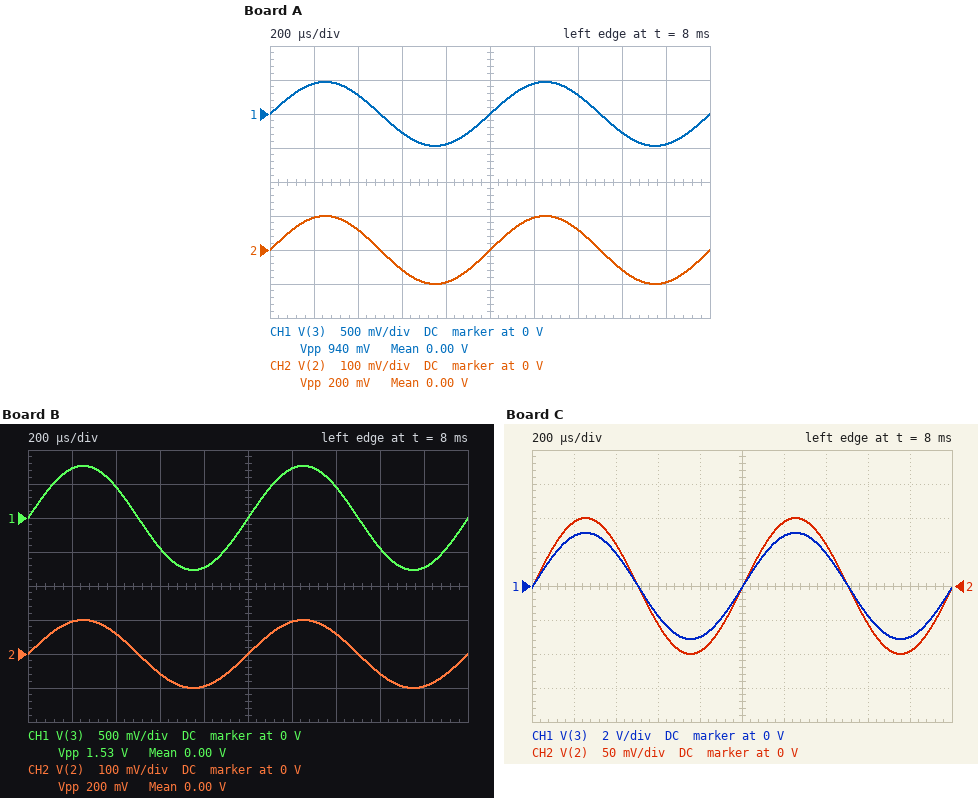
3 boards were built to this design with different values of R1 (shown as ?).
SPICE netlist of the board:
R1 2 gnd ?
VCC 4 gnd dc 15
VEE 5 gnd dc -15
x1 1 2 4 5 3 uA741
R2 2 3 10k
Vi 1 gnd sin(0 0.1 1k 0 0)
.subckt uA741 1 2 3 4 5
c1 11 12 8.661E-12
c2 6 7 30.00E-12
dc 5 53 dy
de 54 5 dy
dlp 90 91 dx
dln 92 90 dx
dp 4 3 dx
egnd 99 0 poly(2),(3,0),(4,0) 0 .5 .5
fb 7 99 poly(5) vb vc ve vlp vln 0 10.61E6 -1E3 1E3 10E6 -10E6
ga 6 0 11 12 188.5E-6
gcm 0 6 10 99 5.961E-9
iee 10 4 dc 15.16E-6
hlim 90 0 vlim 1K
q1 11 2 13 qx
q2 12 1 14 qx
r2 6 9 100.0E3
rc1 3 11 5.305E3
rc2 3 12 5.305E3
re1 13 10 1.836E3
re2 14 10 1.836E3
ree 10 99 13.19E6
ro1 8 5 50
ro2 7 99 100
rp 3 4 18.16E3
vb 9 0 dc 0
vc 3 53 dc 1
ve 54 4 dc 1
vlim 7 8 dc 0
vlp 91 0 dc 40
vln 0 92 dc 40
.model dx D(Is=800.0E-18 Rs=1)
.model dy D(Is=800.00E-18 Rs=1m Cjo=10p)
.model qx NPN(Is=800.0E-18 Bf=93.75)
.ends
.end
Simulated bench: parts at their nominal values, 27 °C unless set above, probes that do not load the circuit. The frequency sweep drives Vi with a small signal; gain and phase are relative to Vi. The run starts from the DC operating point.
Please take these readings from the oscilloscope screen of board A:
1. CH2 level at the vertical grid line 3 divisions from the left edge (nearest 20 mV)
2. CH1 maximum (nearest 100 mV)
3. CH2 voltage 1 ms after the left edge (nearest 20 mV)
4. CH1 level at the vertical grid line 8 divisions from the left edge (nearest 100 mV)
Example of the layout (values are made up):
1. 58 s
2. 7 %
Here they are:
1. -60 mV
2. 500 mV
3. 0 V
4. -300 mV
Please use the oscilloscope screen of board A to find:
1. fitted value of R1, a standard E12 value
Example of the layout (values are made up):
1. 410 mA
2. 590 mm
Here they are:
1. 2.7 kΩ
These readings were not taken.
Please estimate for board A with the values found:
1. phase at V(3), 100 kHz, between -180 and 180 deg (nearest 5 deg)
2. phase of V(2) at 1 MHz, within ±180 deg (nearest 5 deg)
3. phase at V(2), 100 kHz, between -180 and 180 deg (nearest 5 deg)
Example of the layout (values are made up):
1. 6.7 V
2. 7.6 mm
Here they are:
1. -25 deg
2. -110 deg
3. -25 deg
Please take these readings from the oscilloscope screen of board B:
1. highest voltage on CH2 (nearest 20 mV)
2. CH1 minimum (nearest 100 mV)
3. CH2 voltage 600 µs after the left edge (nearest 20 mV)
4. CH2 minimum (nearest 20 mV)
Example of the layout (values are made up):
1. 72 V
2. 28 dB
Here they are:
1. 100 mV
2. -800 mV
3. -60 mV
4. -100 mV
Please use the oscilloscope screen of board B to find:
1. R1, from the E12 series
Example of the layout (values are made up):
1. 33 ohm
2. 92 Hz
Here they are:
1. 1.5 kΩ
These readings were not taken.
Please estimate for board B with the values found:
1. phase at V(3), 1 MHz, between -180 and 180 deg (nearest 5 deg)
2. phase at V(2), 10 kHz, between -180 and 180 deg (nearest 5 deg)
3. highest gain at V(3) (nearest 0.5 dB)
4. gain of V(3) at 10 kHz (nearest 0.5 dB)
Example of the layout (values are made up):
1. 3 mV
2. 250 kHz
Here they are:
1. -115 deg
2. -5 deg
3. 17.5 dB
4. 17.5 dB
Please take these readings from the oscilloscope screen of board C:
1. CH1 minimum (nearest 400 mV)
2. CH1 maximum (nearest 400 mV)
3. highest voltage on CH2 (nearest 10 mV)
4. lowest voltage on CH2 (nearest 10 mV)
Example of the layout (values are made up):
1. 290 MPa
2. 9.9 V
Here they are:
1. -3.2 V
2. 3.2 V
3. 100 mV
4. -100 mV
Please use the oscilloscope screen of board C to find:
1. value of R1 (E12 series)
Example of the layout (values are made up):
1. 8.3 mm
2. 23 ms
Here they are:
1. 330 Ω
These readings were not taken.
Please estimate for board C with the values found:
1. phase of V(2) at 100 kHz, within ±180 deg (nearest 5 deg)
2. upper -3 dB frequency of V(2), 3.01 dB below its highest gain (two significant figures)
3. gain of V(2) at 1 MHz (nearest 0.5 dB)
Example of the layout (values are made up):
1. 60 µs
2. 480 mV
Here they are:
1. -75 deg
2. 32 kHz
3. -31.0 dB
